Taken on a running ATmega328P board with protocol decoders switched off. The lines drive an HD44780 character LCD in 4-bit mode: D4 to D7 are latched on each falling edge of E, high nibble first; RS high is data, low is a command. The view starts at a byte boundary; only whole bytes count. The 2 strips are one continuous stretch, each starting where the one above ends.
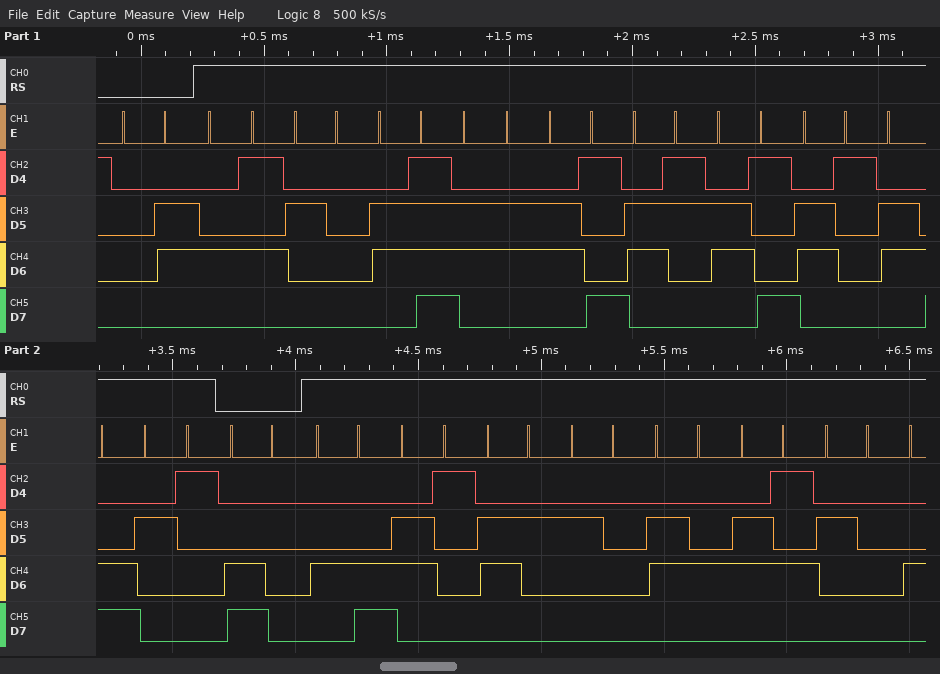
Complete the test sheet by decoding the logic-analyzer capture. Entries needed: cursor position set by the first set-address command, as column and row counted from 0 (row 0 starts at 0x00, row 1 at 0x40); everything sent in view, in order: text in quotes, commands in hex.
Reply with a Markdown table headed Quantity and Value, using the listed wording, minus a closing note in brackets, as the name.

| Quantity | Value |
|---|---|
| cursor position set by the first set-address command, as column and row counted from 0 | column 0, row 1 |
| everything sent in view, in order: text in quotes, commands in hex | 0x06 "E oficial!" 0xC0 "Lab de " |
